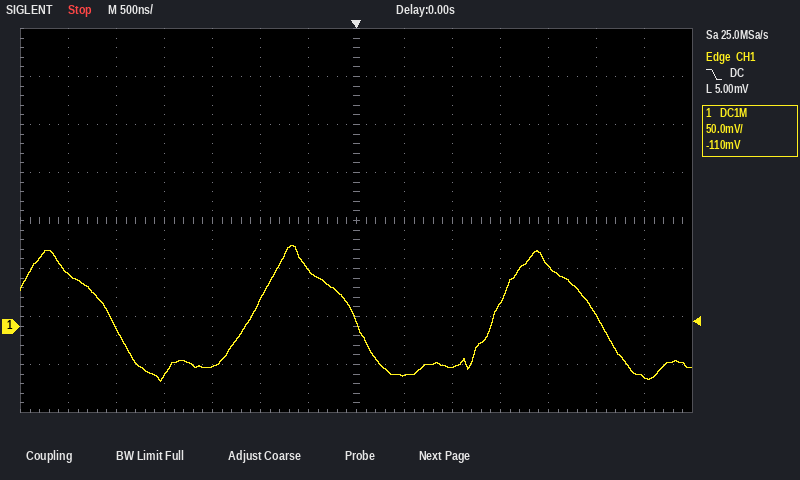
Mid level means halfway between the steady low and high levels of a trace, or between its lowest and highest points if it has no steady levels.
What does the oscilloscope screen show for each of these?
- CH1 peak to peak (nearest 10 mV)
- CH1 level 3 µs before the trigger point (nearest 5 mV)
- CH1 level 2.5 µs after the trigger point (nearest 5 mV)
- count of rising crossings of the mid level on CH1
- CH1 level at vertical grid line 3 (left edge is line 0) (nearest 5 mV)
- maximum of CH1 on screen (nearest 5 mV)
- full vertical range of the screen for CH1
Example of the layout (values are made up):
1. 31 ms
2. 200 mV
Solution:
1. 140 mV
2. 55 mV
3. 10 mV
4. 2
5. -50 mV
6. 85 mV
7. 400 mV
